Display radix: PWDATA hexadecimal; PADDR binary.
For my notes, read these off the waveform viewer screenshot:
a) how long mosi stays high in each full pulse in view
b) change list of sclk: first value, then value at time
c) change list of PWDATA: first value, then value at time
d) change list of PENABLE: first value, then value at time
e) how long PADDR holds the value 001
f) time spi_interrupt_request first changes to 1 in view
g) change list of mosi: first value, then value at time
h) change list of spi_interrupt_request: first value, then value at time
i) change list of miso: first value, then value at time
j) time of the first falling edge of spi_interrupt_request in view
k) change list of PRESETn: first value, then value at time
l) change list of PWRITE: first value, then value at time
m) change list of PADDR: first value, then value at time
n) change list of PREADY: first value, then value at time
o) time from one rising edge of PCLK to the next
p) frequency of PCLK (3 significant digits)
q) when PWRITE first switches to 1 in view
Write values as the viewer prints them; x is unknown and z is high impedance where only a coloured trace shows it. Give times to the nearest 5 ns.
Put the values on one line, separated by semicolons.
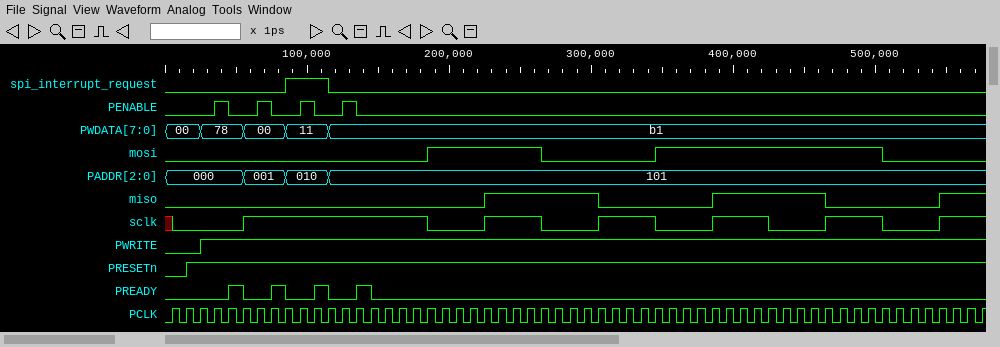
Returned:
80 ns, 160 ns; x, 0 at 5 ns, 1 at 55 ns, 0 at 185 ns, 1 at 225 ns, 0 at 265 ns, 1 at 305 ns, 0 at 345 ns, 1 at 385 ns, 0 at 425 ns, 1 at 465 ns, 0 at 505 ns, 1 at 545 ns; 00, 78 at 25 ns, 00 at 55 ns, 11 at 85 ns, b1 at 115 ns; 0, 1 at 35 ns, 0 at 45 ns, 1 at 65 ns, 0 at 75 ns, 1 at 95 ns, 0 at 105 ns, 1 at 125 ns, 0 at 135 ns; 30 ns; 85 ns; 0, 1 at 185 ns, 0 at 265 ns, 1 at 345 ns, 0 at 505 ns; 0, 1 at 85 ns, 0 at 115 ns; 0, 1 at 225 ns, 0 at 305 ns, 1 at 385 ns, 0 at 465 ns, 1 at 545 ns; 115 ns; 0, 1 at 15 ns; 0, 1 at 25 ns; 000, 001 at 55 ns, 010 at 85 ns, 101 at 115 ns; 0, 1 at 45 ns, 0 at 55 ns, 1 at 75 ns, 0 at 85 ns, 1 at 105 ns, 0 at 115 ns, 1 at 135 ns, 0 at 145 ns; 10 ns; 100 MHz; 25 ns
